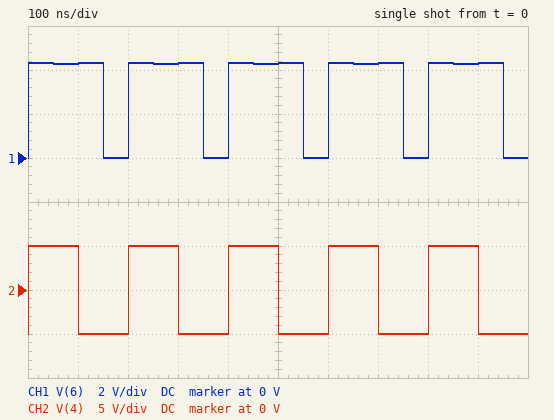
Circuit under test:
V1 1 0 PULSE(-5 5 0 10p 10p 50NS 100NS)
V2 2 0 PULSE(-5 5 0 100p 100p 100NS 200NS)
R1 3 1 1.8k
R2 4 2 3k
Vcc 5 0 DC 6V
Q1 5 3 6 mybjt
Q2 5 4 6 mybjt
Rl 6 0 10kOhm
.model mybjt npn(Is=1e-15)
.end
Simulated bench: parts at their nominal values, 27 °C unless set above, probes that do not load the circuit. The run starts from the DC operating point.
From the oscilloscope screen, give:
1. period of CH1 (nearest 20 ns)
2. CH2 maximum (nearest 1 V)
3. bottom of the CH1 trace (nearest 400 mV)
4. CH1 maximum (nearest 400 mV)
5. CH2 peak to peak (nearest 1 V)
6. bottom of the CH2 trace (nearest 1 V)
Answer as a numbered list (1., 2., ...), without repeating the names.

1. 200 ns
2. 5 V
3. 0 V
4. 4.4 V
5. 10 V
6. -5 V
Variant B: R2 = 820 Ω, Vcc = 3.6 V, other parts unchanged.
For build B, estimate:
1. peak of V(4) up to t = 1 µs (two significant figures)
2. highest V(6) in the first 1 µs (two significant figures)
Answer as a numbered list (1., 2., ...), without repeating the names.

1. 4.3 V
2. 3.6 V
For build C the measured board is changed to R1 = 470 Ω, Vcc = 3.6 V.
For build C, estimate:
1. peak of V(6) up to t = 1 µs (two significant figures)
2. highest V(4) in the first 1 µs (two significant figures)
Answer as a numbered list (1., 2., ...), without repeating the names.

1. 3.6 V
2. 4.3 V
